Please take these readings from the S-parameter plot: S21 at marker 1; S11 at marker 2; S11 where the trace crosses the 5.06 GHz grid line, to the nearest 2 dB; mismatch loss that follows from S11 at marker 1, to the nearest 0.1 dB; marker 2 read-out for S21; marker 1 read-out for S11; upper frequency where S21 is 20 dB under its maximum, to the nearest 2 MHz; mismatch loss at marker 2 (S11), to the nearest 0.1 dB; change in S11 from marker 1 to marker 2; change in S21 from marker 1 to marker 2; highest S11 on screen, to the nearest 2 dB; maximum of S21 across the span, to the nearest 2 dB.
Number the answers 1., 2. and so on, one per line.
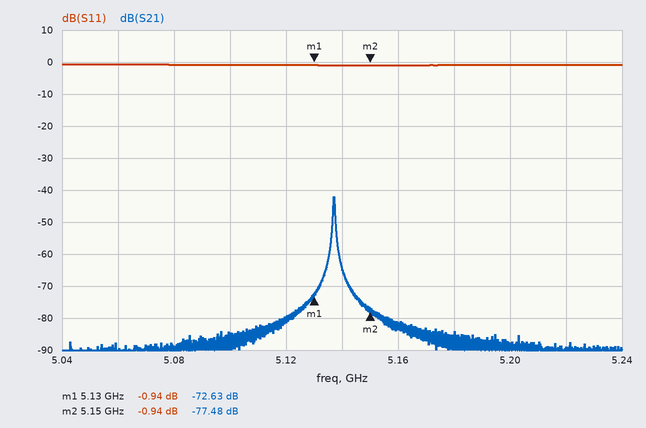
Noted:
1. -72.63 dB
2. -0.94 dB
3. 0 dB
4. 7.1 dB
5. -77.48 dB
6. -0.94 dB
7. 5.140 GHz
8. 7.1 dB
9. 0.00 dB
10. -4.85 dB
11. 0 dB
12. -42 dB
